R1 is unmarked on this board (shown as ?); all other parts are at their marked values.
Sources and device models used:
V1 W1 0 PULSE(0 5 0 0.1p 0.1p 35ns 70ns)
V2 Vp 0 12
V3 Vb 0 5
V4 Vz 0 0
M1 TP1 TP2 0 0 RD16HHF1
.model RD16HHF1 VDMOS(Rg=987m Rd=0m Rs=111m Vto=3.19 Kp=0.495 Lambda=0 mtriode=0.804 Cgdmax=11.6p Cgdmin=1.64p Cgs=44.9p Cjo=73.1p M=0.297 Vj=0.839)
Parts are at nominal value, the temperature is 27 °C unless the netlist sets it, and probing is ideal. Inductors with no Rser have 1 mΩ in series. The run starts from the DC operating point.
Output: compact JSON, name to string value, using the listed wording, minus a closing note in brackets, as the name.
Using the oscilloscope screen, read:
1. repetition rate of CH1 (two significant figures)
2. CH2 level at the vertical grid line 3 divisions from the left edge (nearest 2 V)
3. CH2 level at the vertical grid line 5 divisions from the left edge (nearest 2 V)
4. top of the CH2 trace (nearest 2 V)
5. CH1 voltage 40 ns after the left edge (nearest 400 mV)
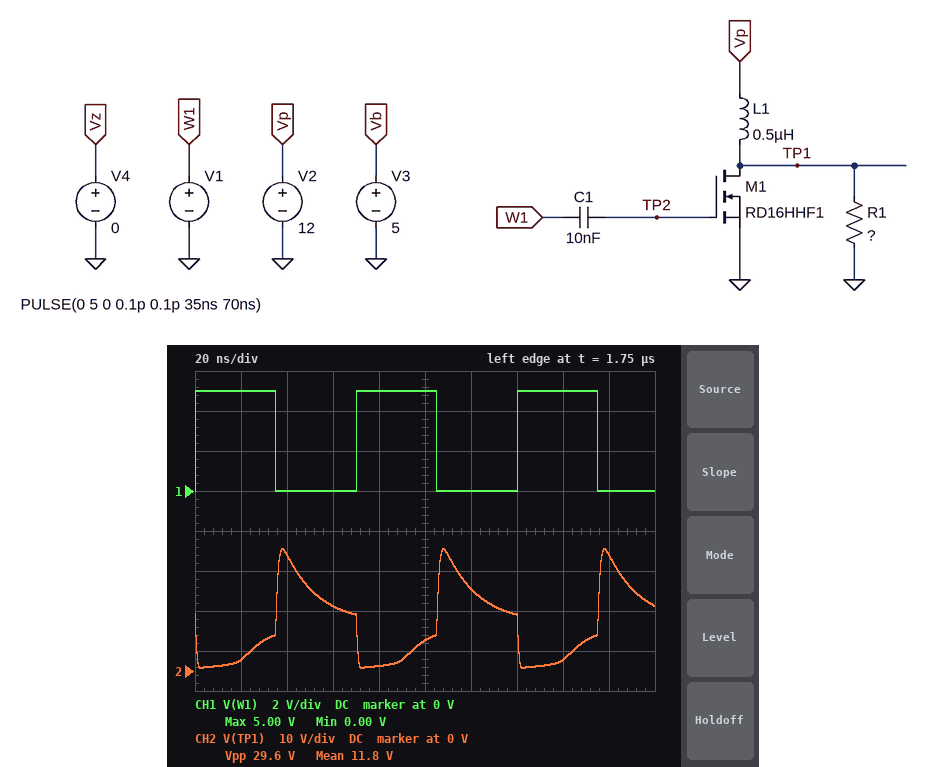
{"repetition rate of CH1": "14 MHz", "CH2 level at the vertical grid line 3 divisions from the left edge": "16 V", "CH2 level at the vertical grid line 5 divisions from the left edge": "8 V", "top of the CH2 trace": "30 V", "CH1 voltage 40 ns after the left edge": "0 V"}
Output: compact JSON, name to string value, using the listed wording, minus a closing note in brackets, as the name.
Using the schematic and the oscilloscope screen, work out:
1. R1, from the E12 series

{"R1, from the E12 series": "33 Ω"}
